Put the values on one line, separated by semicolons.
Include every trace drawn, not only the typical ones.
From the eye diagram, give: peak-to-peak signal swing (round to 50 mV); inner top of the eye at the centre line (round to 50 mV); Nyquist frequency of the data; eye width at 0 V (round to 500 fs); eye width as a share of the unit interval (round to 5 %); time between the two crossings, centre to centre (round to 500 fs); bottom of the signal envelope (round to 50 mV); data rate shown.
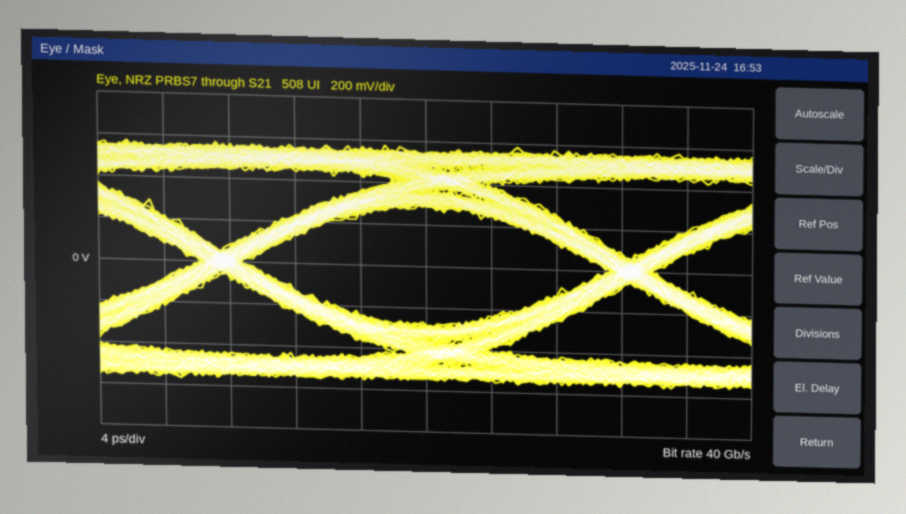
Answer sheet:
1.15 V; 300 mV; 20 GHz; 22.5 ps; 90 %; 25.0 ps; -550 mV; 40 Gb/s
